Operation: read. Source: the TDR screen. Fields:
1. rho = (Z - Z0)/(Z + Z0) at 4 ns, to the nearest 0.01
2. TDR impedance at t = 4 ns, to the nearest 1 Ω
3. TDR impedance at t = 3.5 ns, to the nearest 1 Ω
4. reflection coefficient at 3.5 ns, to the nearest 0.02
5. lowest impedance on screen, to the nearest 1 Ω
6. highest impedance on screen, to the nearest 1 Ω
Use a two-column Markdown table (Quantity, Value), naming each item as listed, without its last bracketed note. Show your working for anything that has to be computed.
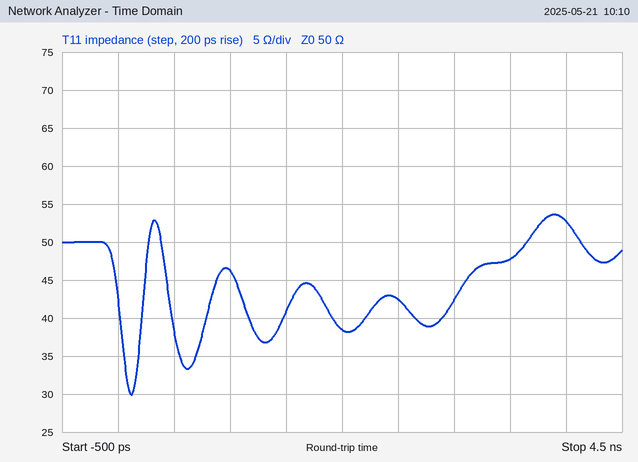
| Quantity | Value |
|---|---|
| rho = (Z - Z0)/(Z + Z0) at 4 ns, to the nearest 0.01 | (53 − 50)/(53 + 50) ≈ +0.03 |
| TDR impedance at t = 4 ns, to the nearest 1 Ω | 53 Ω |
| TDR impedance at t = 3.5 ns, to the nearest 1 Ω | 48 Ω |
| reflection coefficient at 3.5 ns, to the nearest 0.02 | (48 − 50)/(48 + 50) ≈ -0.02 |
| lowest impedance on screen, to the nearest 1 Ω | 30 Ω |
| highest impedance on screen, to the nearest 1 Ω | 54 Ω |
